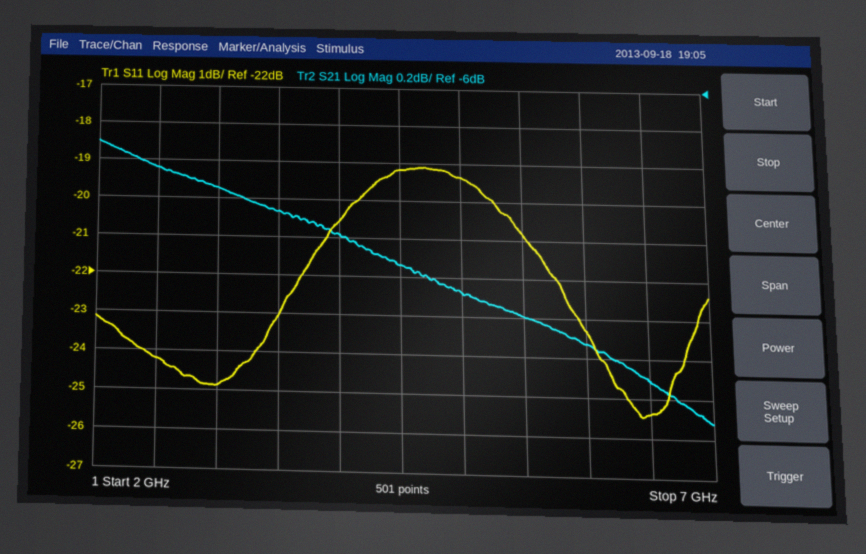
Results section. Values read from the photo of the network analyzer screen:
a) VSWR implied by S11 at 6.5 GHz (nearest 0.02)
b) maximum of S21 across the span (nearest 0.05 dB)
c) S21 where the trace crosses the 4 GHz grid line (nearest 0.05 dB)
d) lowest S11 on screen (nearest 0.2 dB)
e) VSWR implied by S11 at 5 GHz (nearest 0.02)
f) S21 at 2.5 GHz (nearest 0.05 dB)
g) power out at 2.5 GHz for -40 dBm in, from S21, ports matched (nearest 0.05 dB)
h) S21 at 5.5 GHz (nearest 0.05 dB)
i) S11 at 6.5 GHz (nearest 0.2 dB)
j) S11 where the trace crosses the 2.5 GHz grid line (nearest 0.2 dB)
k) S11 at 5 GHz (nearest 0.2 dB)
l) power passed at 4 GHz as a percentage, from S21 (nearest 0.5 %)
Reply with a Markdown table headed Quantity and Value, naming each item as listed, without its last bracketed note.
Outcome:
| Quantity | Value |
|---|---|
| VSWR implied by S11 at 6.5 GHz | 1.12 |
| maximum of S21 across the span | -6.30 dB |
| S21 where the trace crosses the 4 GHz grid line | -6.80 dB |
| lowest S11 on screen | -25.4 dB |
| VSWR implied by S11 at 5 GHz | 1.24 |
| S21 at 2.5 GHz | -6.45 dB |
| power out at 2.5 GHz for -40 dBm in, from S21, ports matched | -46.45 dBm |
| S21 at 5.5 GHz | -7.20 dB |
| S11 at 6.5 GHz | -25.4 dB |
| S11 where the trace crosses the 2.5 GHz grid line | -24.2 dB |
| S11 at 5 GHz | -19.4 dB |
| power passed at 4 GHz as a percentage, from S21 | 21.0 % |
